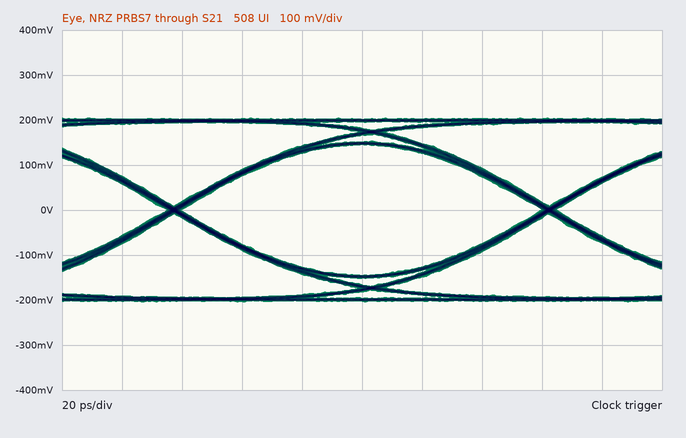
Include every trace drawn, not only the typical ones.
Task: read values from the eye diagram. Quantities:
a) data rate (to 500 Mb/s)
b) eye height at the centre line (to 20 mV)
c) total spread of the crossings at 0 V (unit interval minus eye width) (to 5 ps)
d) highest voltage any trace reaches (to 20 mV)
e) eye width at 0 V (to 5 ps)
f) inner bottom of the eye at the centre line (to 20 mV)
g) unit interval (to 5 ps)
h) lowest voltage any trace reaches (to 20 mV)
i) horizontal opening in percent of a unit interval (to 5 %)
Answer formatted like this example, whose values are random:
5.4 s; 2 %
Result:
8.0 Gb/s; 300 mV; 5 ps; 200 mV; 120 ps; -140 mV; 125 ps; -200 mV; 95 %
